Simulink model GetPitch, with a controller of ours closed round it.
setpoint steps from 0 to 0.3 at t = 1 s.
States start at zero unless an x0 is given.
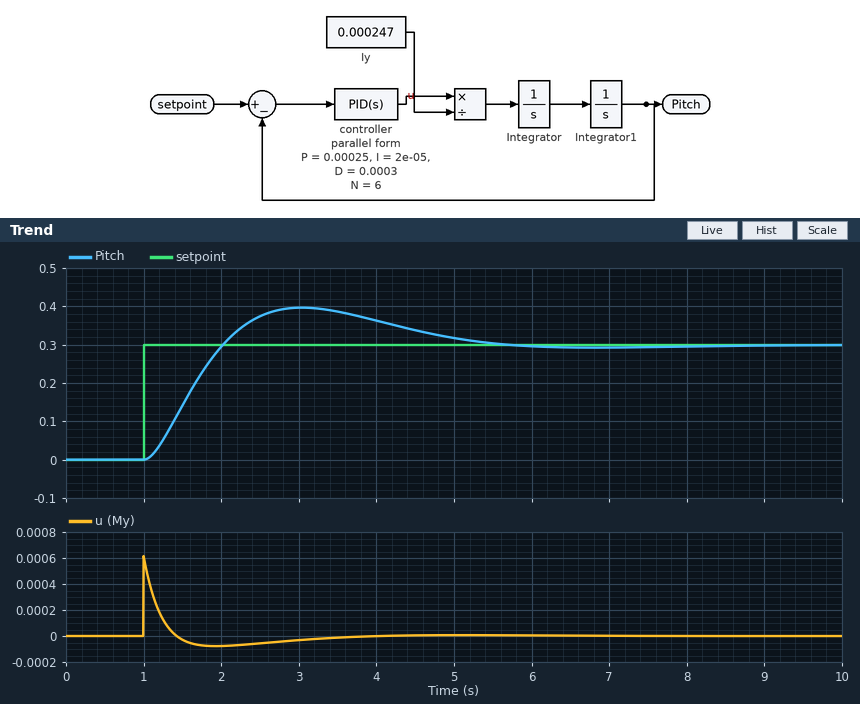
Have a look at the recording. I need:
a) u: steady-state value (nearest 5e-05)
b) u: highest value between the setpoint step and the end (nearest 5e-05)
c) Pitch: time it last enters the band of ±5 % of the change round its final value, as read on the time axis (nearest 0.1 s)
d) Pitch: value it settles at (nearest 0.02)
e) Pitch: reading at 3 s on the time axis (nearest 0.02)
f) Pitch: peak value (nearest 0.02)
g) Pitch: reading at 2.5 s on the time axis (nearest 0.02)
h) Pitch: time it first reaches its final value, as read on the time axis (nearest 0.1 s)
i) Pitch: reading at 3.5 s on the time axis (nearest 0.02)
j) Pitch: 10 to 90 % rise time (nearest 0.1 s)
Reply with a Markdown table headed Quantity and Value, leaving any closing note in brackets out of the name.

| Quantity | Value |
|---|---|
| u: steady-state value | 0.00000 |
| u: highest value between the setpoint step and the end | 0.00060 |
| Pitch: time it last enters the band of ±5 % of the change round its final value, as read on the time axis | 5.1 s |
| Pitch: value it settles at | 0.30 |
| Pitch: reading at 3 s on the time axis | 0.40 |
| Pitch: peak value | 0.40 |
| Pitch: reading at 2.5 s on the time axis | 0.38 |
| Pitch: time it first reaches its final value, as read on the time axis | 2.0 s |
| Pitch: reading at 3.5 s on the time axis | 0.38 |
| Pitch: 10 to 90 % rise time | 0.7 s |
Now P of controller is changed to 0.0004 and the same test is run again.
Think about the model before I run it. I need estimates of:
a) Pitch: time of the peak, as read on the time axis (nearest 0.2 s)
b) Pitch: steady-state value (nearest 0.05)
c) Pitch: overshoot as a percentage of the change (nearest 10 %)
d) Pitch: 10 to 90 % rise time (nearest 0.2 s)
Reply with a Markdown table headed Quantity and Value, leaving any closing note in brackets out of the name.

| Quantity | Value |
|---|---|
| Pitch: time of the peak, as read on the time axis | 2.8 s |
| Pitch: steady-state value | 0.30 |
| Pitch: overshoot as a percentage of the change | 40 % |
| Pitch: 10 to 90 % rise time | 0.6 s |
